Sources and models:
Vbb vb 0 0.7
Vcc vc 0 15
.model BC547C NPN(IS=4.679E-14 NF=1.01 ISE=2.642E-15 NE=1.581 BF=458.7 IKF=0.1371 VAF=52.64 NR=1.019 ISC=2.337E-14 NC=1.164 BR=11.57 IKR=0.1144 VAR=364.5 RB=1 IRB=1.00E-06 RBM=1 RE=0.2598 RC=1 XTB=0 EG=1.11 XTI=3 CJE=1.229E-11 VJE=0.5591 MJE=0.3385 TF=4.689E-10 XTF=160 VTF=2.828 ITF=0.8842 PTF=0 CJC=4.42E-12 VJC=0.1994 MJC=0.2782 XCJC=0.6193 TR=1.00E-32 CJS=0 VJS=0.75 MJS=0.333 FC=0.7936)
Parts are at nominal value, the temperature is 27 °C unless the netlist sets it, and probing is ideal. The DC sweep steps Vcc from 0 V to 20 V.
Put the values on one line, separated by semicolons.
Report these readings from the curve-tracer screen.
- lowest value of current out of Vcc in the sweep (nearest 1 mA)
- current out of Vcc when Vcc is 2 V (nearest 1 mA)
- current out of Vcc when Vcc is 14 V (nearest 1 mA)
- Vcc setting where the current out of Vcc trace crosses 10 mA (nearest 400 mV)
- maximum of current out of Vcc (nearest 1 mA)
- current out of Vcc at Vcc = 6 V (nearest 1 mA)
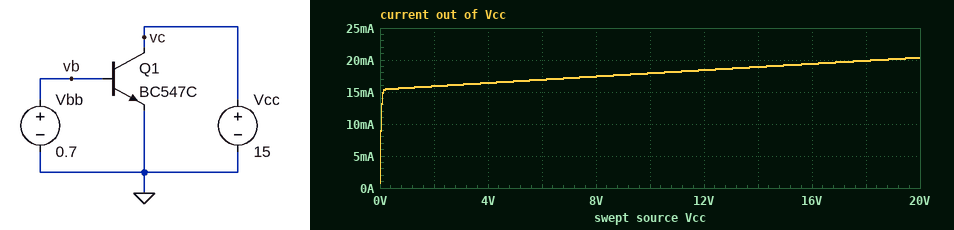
1 mA; 16 mA; 19 mA; 0 V; 20 mA; 17 mA
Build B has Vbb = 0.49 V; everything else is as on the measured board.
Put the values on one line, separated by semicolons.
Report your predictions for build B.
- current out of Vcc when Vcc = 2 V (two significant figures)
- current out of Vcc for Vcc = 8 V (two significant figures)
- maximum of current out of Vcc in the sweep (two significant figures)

6.7 µA; 7.5 µA; 9.0 µA
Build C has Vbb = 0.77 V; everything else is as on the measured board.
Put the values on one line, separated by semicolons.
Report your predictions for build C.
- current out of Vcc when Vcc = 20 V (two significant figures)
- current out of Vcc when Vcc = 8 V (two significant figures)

98 mA; 88 mA
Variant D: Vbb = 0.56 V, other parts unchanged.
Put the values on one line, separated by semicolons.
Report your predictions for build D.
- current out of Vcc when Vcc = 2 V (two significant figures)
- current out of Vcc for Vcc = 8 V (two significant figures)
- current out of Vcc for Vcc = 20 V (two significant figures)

98 µA; 110 µA; 130 µA
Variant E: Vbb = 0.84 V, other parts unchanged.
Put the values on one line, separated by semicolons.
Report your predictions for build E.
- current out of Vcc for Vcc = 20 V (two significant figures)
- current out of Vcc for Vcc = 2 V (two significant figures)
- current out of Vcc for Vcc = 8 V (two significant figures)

240 mA; 210 mA; 220 mA
